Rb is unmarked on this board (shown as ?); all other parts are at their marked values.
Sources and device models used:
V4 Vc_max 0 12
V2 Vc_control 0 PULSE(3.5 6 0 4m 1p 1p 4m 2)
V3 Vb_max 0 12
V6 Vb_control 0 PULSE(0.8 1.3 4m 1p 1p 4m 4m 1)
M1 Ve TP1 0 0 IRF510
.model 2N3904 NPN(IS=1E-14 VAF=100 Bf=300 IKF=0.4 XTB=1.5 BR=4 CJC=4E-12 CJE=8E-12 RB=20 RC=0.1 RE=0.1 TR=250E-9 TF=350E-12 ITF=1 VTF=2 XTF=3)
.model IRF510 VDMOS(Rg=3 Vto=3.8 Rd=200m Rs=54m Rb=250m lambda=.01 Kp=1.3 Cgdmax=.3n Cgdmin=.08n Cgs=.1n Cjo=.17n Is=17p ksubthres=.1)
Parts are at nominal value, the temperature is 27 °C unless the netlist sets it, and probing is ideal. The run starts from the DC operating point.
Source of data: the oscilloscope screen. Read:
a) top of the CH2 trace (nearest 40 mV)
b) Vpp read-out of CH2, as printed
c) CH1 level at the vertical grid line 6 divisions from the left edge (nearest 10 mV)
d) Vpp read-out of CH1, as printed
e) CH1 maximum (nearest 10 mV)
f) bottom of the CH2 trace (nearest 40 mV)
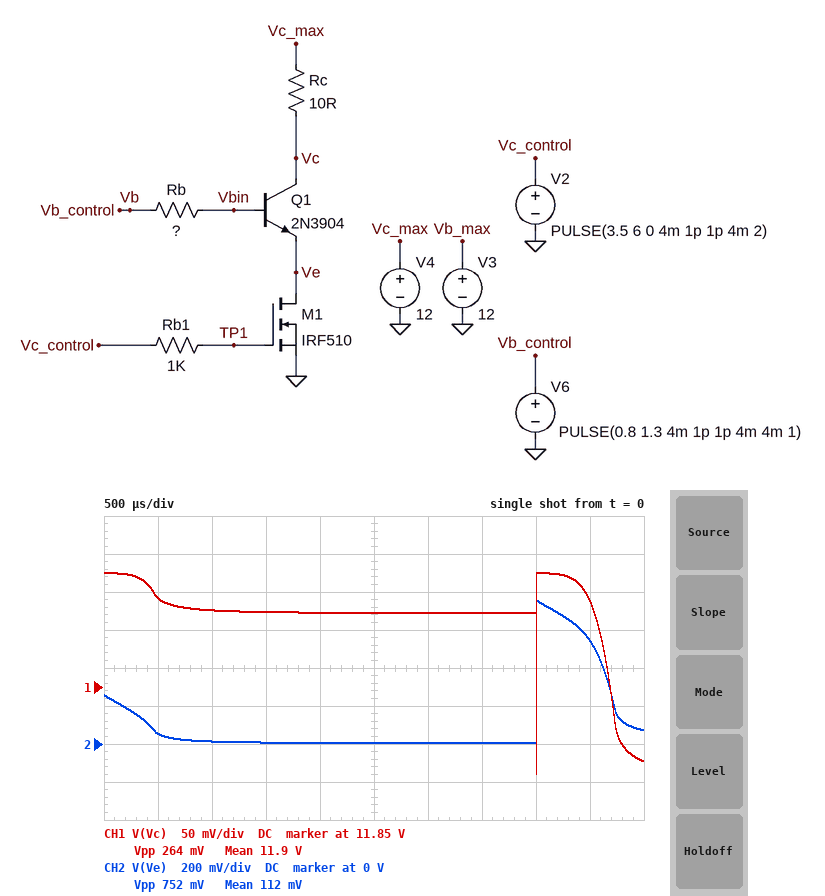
760 mV
752 mV
11.95 V
264 mV
12.00 V
0 V
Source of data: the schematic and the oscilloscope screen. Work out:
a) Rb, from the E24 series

6.2 kΩ
